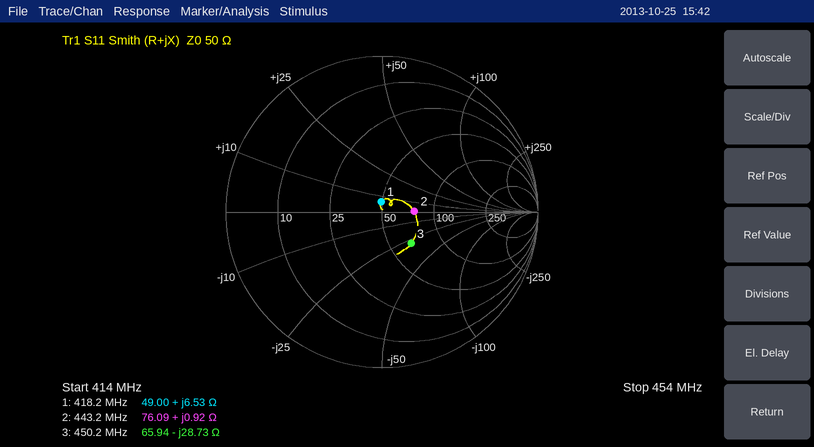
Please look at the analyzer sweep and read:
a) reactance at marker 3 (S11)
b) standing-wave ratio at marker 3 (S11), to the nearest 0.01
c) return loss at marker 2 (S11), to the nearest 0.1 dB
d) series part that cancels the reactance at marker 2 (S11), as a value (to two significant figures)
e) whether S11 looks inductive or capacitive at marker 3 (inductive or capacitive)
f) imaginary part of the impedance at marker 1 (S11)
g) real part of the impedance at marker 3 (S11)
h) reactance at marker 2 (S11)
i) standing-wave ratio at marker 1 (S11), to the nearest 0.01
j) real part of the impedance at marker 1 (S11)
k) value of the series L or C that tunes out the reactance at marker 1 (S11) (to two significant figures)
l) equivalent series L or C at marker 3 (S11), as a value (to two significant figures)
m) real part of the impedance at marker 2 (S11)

-28.73 Ω
1.76
13.7 dB
390 pF
capacitive
+6.53 Ω
65.94 Ω
+0.92 Ω
1.14
49.00 Ω
58 pF
12 pF
76.09 Ω
